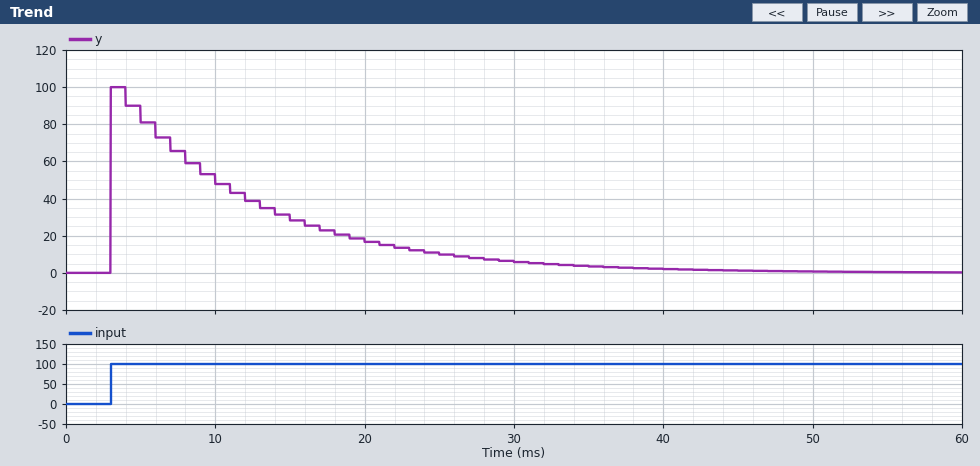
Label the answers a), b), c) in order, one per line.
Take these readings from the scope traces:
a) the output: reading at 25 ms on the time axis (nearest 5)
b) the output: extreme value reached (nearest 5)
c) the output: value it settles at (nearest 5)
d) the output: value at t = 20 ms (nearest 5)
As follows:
a) 10
b) 100
c) 0
d) 15
